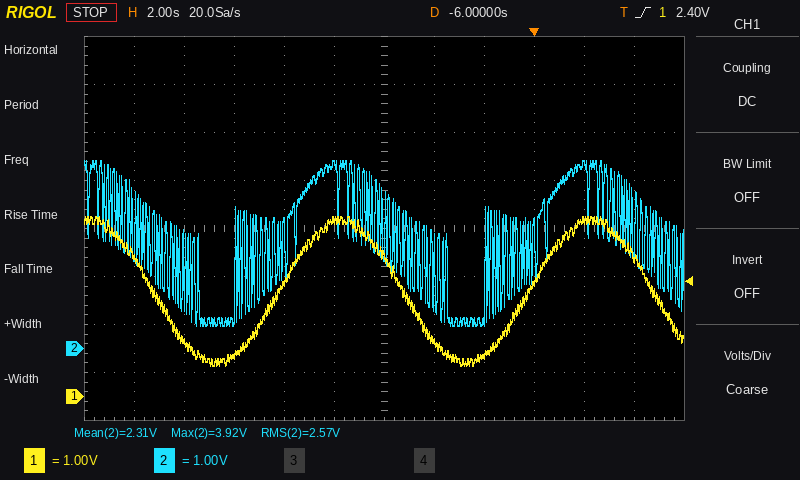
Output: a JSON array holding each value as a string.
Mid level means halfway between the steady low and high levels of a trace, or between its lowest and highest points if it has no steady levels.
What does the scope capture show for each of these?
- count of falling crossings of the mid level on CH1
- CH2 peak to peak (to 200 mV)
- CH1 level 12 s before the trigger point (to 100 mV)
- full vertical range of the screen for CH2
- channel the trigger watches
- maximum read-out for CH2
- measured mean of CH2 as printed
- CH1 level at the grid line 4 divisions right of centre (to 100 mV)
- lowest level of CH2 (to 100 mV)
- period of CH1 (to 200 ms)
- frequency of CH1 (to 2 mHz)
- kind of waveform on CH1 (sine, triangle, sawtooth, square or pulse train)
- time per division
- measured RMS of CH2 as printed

["3", "3.4 V", "900 mV", "8 V", "CH1", "3.92 V", "2.31 V", "3.7 V", "500 mV", "10.0 s", "100 mHz", "sine", "2 s", "2.57 V"]
